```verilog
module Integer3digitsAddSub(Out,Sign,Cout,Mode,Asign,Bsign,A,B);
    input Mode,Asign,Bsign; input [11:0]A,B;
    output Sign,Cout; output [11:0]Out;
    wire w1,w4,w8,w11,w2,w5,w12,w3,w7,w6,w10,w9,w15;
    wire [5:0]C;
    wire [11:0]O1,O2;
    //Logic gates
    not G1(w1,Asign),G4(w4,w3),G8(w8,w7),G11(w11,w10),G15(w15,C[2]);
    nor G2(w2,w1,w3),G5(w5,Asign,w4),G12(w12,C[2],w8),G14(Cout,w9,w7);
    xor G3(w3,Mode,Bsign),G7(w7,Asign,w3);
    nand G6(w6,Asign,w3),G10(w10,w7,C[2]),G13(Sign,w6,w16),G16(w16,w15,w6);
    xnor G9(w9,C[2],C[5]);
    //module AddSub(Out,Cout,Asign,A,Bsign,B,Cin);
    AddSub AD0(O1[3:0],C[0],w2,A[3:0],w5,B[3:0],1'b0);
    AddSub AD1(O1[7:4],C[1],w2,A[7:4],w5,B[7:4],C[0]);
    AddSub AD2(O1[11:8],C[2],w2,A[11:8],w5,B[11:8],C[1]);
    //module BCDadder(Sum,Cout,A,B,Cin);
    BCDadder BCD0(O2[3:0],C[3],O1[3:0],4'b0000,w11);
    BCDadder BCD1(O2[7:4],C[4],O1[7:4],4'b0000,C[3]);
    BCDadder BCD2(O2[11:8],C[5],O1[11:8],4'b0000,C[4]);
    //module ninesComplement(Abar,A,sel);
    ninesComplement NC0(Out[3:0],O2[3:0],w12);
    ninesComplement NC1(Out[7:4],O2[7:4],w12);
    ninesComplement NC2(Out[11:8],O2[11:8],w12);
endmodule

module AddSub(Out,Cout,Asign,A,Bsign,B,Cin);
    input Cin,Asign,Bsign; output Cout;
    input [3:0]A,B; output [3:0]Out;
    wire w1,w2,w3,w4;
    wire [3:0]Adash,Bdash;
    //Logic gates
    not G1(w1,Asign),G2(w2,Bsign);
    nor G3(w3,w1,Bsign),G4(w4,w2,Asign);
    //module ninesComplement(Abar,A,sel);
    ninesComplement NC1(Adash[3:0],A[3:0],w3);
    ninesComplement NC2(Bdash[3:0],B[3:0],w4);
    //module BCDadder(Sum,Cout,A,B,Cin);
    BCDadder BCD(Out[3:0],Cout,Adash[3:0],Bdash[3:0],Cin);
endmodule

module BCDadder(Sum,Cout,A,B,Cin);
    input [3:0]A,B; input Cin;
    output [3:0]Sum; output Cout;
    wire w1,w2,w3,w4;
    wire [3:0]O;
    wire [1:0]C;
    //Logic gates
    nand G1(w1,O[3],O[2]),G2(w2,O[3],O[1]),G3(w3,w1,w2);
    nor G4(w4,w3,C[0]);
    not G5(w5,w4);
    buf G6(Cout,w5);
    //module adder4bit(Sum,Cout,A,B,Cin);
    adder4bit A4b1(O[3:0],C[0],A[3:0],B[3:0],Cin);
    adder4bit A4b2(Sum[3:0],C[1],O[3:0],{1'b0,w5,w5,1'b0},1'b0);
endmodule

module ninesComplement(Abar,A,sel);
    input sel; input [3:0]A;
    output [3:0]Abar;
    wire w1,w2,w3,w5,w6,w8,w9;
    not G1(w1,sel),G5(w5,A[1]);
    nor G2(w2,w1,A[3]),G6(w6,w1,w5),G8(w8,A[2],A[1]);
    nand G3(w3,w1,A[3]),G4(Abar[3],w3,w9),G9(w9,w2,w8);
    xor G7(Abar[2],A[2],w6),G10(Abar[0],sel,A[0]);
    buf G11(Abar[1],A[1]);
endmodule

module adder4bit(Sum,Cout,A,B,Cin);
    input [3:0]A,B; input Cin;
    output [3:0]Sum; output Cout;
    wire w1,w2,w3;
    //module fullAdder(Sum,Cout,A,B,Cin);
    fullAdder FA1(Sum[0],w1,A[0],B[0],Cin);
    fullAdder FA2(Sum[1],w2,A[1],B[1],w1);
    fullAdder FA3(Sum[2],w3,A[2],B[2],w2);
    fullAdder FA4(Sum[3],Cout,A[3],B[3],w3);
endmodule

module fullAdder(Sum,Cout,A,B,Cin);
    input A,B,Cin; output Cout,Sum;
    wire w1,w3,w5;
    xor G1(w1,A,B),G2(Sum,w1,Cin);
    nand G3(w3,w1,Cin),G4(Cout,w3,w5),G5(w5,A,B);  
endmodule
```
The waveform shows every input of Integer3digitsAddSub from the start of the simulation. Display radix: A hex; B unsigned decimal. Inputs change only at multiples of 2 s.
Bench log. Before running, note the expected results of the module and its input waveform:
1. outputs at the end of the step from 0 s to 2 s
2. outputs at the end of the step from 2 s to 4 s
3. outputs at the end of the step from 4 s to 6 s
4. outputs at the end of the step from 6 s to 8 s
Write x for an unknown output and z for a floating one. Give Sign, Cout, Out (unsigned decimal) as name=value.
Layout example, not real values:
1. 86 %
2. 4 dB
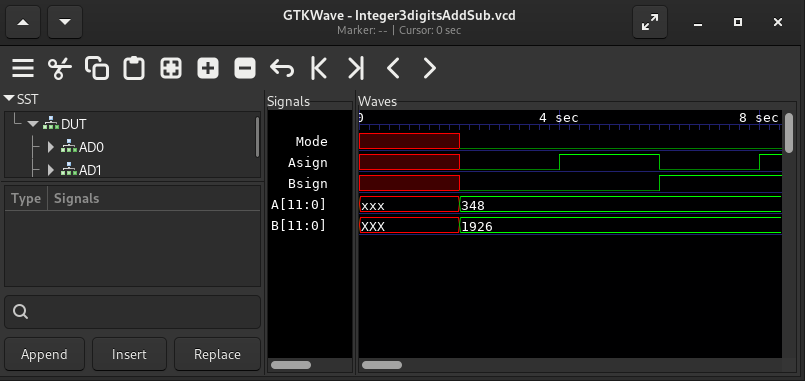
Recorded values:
1. Sign=x, Cout=x, Out=x
2. Sign=0, Cout=1, Out=308
3. Sign=0, Cout=0, Out=1080
4. Sign=1, Cout=0, Out=1080
